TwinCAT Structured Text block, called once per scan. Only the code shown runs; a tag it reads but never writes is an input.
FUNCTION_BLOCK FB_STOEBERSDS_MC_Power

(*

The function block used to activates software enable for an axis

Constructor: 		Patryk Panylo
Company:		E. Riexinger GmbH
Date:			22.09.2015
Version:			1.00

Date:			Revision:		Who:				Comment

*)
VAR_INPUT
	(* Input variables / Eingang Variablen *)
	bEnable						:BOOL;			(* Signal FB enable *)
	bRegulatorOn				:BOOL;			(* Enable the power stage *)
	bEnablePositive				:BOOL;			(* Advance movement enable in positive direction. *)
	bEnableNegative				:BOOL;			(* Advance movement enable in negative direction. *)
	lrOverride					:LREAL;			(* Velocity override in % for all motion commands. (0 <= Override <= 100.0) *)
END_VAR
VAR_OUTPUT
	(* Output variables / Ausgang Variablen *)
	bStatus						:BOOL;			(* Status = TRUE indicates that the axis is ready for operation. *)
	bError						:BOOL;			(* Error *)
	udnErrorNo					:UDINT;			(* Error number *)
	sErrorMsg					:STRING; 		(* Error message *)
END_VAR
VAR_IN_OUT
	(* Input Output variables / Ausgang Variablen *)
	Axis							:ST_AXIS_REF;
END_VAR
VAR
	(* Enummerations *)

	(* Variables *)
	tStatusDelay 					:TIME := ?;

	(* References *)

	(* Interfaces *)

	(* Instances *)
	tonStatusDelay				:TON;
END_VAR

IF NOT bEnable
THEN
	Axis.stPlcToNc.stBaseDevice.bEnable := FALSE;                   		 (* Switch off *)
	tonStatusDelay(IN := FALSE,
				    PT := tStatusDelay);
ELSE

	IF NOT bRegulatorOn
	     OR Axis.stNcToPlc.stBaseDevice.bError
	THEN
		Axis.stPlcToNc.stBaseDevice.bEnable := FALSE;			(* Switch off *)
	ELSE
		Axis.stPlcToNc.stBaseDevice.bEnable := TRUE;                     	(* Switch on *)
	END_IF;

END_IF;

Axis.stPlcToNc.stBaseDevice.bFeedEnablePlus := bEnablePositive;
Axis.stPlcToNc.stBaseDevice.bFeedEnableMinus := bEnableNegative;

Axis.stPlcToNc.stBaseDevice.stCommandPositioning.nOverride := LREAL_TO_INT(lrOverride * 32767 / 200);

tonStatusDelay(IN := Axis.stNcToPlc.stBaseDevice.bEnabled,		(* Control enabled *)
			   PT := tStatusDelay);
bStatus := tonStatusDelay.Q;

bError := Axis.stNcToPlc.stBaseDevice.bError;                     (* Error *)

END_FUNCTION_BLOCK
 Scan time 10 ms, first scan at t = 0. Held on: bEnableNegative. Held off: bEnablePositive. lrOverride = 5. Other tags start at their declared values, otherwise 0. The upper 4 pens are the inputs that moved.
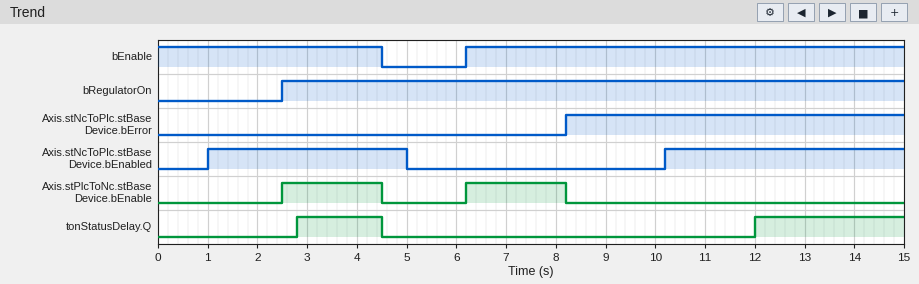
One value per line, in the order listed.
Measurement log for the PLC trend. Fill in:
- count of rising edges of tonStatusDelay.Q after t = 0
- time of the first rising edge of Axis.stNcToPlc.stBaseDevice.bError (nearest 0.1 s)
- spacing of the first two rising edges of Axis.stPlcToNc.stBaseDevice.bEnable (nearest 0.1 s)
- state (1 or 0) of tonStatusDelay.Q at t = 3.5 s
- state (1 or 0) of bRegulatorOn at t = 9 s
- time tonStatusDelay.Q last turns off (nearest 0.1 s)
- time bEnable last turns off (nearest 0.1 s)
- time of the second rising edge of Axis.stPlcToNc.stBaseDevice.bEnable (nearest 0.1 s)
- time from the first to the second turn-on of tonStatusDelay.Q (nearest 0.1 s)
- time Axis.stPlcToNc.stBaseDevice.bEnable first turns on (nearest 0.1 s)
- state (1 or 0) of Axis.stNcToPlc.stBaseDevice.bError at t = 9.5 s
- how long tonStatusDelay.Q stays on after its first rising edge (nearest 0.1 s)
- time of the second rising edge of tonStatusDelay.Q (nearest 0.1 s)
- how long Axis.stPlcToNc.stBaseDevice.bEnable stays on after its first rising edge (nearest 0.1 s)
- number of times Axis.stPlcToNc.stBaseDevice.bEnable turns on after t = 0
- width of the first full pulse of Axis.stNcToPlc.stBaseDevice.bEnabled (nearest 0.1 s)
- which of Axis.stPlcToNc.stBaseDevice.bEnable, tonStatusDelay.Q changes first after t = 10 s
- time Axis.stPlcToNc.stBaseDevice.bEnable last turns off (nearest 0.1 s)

2
8.2 s
3.7 s
1
1
4.5 s
4.5 s
6.2 s
9.2 s
2.5 s
1
1.7 s
12.0 s
2.0 s
2
4.0 s
tonStatusDelay.Q
8.2 s
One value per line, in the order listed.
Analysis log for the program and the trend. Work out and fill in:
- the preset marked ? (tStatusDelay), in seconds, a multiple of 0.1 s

1.8 s
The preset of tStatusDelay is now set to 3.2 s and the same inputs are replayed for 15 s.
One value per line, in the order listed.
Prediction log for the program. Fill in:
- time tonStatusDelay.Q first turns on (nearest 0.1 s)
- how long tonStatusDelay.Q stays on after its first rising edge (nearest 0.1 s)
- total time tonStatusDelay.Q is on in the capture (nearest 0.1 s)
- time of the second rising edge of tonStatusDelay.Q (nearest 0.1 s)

4.2 s
0.3 s
1.9 s
13.4 s
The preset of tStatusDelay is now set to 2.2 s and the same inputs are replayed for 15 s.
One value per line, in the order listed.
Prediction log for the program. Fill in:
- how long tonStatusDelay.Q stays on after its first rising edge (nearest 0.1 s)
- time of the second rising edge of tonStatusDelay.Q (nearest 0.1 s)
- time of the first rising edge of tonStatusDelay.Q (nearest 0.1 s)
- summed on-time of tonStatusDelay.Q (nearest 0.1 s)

1.3 s
12.4 s
3.2 s
3.9 s
